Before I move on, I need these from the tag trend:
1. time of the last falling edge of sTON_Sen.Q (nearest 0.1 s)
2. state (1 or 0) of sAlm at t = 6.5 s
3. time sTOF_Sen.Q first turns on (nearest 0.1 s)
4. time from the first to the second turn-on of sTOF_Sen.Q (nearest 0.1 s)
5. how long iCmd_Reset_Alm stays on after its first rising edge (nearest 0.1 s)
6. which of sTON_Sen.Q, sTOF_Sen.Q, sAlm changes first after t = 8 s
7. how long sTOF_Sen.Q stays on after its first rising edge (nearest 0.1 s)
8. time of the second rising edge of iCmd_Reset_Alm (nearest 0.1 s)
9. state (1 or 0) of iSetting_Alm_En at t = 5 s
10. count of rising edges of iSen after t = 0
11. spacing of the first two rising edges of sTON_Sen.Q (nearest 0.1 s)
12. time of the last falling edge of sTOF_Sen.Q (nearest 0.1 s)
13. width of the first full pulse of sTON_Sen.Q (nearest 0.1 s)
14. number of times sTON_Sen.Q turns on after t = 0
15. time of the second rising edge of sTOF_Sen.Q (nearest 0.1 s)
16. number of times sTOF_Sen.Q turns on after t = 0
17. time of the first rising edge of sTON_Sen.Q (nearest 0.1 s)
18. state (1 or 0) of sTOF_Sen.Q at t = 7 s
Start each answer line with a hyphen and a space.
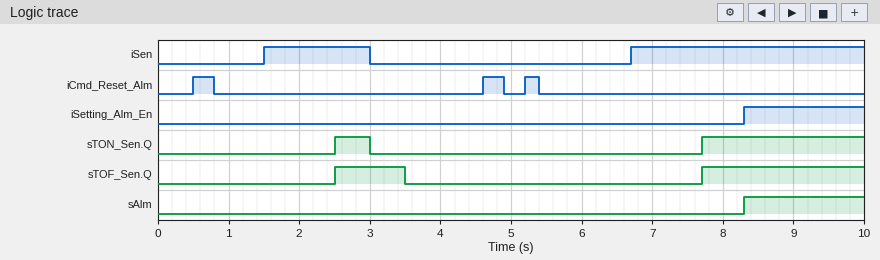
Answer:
- 3.0 s
- 0
- 2.5 s
- 5.2 s
- 0.3 s
- sAlm
- 1.0 s
- 4.6 s
- 0
- 2
- 5.2 s
- 3.5 s
- 0.5 s
- 2
- 7.7 s
- 2
- 2.5 s
- 0
